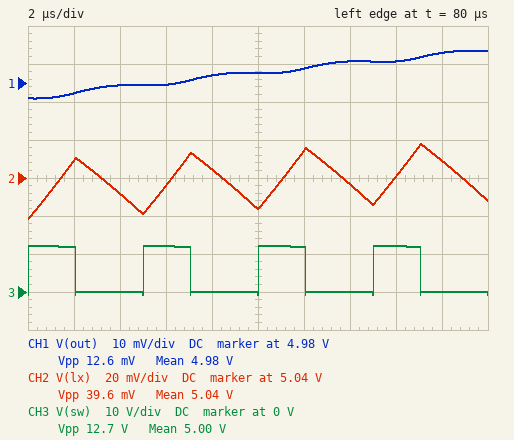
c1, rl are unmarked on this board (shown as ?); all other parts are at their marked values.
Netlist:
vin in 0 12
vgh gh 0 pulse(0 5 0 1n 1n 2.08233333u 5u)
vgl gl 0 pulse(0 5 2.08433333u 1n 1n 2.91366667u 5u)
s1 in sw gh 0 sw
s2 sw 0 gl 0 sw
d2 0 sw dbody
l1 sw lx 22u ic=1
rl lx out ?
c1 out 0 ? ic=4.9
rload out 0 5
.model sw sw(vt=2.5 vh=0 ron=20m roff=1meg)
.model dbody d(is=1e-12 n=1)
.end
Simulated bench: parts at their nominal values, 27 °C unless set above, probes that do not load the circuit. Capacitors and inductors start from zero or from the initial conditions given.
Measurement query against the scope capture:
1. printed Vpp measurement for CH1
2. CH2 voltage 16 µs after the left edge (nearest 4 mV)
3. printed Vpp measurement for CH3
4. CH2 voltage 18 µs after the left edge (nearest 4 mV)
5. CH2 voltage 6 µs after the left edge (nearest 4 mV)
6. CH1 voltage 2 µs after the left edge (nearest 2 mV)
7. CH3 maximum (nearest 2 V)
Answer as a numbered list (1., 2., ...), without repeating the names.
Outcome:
1. 12.6 mV
2. 5.040 V
3. 12.7 V
4. 5.048 V
5. 5.036 V
6. 4.978 V
7. 12 V
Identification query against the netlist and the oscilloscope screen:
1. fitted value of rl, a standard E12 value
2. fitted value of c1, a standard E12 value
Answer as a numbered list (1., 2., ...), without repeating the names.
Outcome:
1. 0.047 Ω
2. 330 µF
